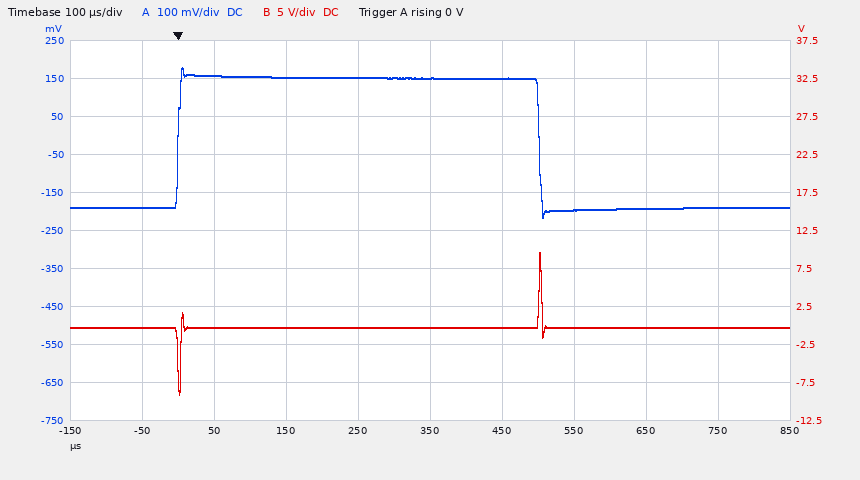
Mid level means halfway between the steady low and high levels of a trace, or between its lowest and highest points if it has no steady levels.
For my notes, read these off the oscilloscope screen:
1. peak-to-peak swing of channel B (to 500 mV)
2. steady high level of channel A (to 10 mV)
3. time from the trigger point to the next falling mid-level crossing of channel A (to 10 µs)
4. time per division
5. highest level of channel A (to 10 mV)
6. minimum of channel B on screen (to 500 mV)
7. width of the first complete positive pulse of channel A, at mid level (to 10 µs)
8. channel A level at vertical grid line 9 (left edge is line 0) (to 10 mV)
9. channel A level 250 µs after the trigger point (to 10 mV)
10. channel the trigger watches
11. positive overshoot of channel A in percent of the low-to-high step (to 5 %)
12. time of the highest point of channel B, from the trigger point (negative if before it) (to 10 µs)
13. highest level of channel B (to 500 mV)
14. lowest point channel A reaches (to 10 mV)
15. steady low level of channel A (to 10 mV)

18.5 V
150 mV
500 µs
100 µs
180 mV
-9.0 V
500 µs
-190 mV
150 mV
channel A
10 %
+500 µs
9.5 V
-220 mV
-190 mV
